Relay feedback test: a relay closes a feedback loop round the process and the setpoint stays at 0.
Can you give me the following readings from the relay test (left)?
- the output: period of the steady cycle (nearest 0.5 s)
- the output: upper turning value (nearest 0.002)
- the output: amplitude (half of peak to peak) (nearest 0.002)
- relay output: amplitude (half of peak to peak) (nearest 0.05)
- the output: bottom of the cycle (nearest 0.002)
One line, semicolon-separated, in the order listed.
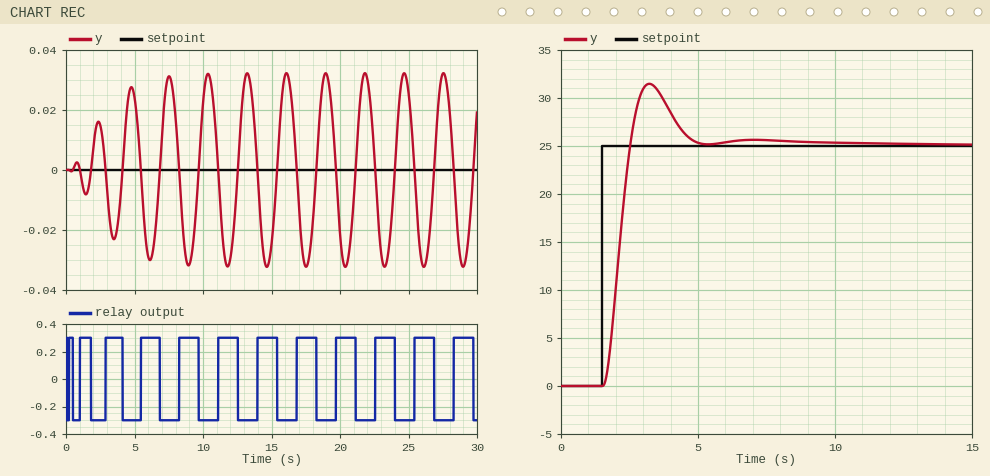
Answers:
3.0 s; 0.032; 0.032; 0.30; -0.032
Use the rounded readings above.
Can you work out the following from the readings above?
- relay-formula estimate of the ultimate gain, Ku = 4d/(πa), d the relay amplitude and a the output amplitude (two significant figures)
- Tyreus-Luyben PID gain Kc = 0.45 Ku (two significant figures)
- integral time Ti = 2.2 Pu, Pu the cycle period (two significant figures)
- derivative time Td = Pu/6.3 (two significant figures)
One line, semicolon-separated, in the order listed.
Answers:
12; 5.4; 6.6 s; 0.48 s
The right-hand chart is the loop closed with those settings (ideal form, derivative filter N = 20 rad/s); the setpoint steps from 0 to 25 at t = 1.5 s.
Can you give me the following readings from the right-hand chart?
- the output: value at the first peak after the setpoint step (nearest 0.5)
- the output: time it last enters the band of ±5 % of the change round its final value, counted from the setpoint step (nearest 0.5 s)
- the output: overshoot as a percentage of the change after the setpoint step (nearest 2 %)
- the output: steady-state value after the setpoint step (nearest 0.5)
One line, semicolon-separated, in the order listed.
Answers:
31.5; 3.0 s; 26 %; 25.0
